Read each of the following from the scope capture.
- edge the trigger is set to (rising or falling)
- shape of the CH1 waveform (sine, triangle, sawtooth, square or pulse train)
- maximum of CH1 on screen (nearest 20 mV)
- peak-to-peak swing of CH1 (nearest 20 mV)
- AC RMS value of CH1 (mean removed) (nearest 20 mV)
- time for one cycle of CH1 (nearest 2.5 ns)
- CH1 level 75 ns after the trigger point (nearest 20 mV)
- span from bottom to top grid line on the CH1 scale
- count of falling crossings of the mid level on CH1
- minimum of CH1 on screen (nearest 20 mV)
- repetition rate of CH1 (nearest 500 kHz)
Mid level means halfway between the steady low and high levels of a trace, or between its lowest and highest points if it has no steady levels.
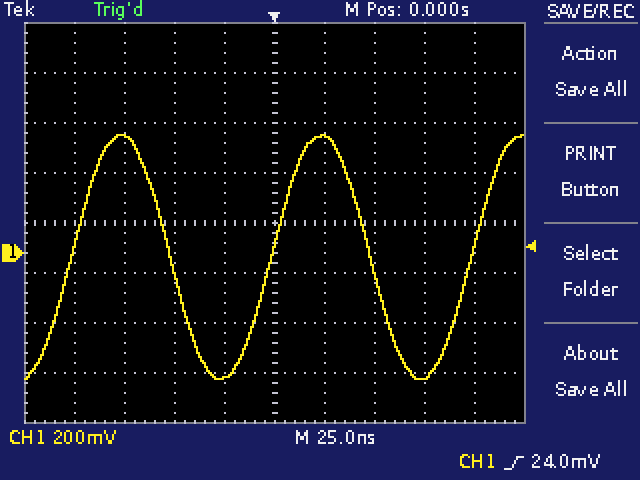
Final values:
rising
sine
480 mV
980 mV
340 mV
100.0 ns
-500 mV
1.6 V
2
-500 mV
10.0 MHz
